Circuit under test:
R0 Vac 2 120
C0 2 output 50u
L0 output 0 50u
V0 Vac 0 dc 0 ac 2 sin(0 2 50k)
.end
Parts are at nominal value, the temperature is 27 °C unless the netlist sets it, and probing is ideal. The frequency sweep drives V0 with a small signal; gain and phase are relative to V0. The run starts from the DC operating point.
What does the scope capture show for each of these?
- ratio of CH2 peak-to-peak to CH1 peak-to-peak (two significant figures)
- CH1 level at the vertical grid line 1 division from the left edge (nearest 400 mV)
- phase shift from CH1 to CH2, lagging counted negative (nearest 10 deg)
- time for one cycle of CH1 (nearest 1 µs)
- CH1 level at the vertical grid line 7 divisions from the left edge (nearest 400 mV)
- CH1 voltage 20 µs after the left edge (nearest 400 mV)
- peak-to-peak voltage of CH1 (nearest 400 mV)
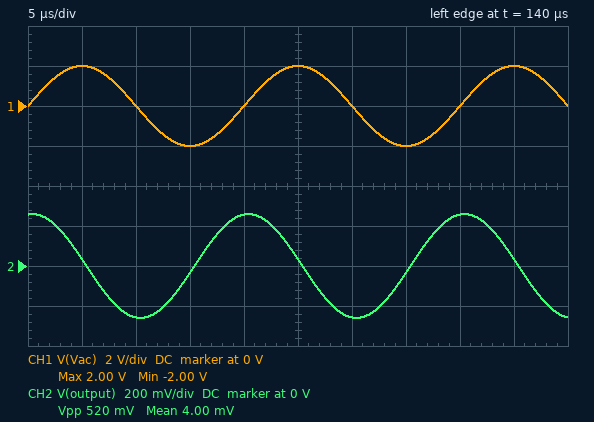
0.13
2.0 V
80 deg
20 µs
-2.0 V
0 V
4.0 V
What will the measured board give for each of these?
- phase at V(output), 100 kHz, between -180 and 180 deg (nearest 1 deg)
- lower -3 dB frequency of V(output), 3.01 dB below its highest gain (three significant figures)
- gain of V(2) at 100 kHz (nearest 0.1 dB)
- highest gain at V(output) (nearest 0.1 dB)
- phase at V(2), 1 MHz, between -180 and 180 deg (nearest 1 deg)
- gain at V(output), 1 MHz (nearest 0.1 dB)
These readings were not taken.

75 deg
382 kHz
-11.9 dB
0 dB
21 deg
-0.6 dB
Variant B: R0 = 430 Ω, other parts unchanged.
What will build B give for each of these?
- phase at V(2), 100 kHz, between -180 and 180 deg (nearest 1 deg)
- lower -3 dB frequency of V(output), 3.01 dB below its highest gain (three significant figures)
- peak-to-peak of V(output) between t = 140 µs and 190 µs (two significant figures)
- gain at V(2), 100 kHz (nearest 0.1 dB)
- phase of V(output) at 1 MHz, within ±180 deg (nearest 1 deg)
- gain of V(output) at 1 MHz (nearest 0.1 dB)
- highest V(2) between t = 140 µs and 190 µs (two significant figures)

86 deg
1.37 MHz
150 mV
-22.8 dB
54 deg
-4.6 dB
73 mV
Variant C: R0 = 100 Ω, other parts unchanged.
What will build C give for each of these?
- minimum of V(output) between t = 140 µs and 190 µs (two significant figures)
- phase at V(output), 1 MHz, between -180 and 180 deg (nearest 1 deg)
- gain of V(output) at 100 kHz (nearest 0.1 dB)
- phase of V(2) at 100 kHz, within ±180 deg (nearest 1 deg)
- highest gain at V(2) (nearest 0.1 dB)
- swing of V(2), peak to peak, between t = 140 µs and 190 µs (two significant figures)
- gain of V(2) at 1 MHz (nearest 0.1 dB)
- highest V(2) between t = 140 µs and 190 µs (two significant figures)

-310 mV
18 deg
-10.5 dB
73 deg
0 dB
620 mV
-0.4 dB
310 mV
